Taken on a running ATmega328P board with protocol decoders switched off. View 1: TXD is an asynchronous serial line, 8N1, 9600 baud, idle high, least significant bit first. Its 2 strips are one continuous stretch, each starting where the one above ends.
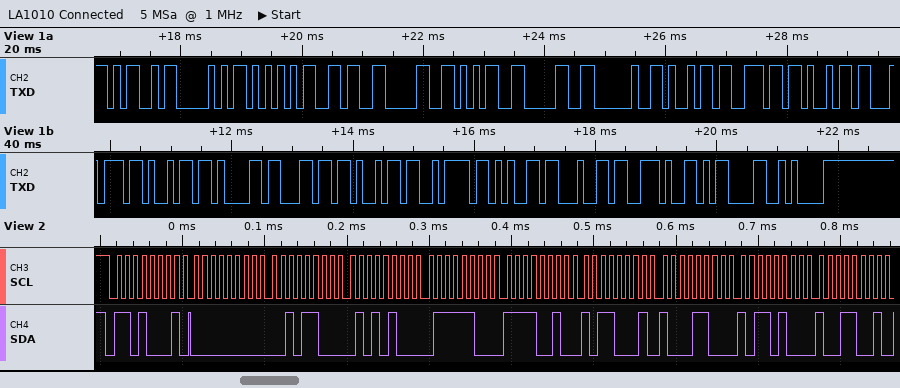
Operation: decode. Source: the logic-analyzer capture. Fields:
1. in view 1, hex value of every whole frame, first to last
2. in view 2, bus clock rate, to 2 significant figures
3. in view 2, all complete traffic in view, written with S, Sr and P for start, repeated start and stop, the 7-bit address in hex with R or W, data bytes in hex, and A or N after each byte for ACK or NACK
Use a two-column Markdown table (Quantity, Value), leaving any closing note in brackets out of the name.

| Quantity | Value |
|---|---|
| in view 1, hex value of every whole frame, first to last | 0x4D 0x50 0x55 0x36 0x30 0x35 0x30 0x20 0x69 0x6E 0x69 0x74 0x69 0x61 0x6C 0x69 0x7A 0x65 0x64 0x2E 0x0D 0x0A |
| in view 2, bus clock rate, to 2 significant figures | 100 kHz |
| in view 2, all complete traffic in view, written with S, Sr and P for start, repeated start and stop, the 7-bit address in hex with R or W, data bytes in hex, and A or N after each byte for ACK or NACK | S 68R A 00 A 2C A 54 A 7C A F2 A B1 A 8C A B4 A 99 A |
